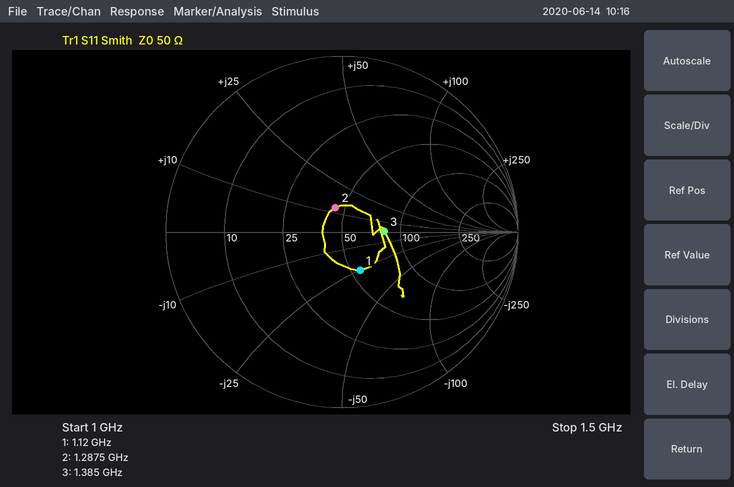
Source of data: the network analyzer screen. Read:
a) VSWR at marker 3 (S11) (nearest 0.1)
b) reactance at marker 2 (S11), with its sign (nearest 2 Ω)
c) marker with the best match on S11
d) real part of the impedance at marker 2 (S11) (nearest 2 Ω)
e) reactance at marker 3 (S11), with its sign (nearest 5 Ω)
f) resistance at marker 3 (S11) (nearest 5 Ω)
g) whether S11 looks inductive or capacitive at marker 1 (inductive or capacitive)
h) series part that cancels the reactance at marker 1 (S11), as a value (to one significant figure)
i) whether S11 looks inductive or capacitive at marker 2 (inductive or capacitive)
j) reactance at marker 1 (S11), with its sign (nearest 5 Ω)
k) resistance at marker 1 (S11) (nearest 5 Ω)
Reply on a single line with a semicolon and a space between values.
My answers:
1.6; +12 Ω; marker 2; 44 Ω; 0 Ω; 80 Ω; capacitive; 4 nH; inductive; -25 Ω; 55 Ω
